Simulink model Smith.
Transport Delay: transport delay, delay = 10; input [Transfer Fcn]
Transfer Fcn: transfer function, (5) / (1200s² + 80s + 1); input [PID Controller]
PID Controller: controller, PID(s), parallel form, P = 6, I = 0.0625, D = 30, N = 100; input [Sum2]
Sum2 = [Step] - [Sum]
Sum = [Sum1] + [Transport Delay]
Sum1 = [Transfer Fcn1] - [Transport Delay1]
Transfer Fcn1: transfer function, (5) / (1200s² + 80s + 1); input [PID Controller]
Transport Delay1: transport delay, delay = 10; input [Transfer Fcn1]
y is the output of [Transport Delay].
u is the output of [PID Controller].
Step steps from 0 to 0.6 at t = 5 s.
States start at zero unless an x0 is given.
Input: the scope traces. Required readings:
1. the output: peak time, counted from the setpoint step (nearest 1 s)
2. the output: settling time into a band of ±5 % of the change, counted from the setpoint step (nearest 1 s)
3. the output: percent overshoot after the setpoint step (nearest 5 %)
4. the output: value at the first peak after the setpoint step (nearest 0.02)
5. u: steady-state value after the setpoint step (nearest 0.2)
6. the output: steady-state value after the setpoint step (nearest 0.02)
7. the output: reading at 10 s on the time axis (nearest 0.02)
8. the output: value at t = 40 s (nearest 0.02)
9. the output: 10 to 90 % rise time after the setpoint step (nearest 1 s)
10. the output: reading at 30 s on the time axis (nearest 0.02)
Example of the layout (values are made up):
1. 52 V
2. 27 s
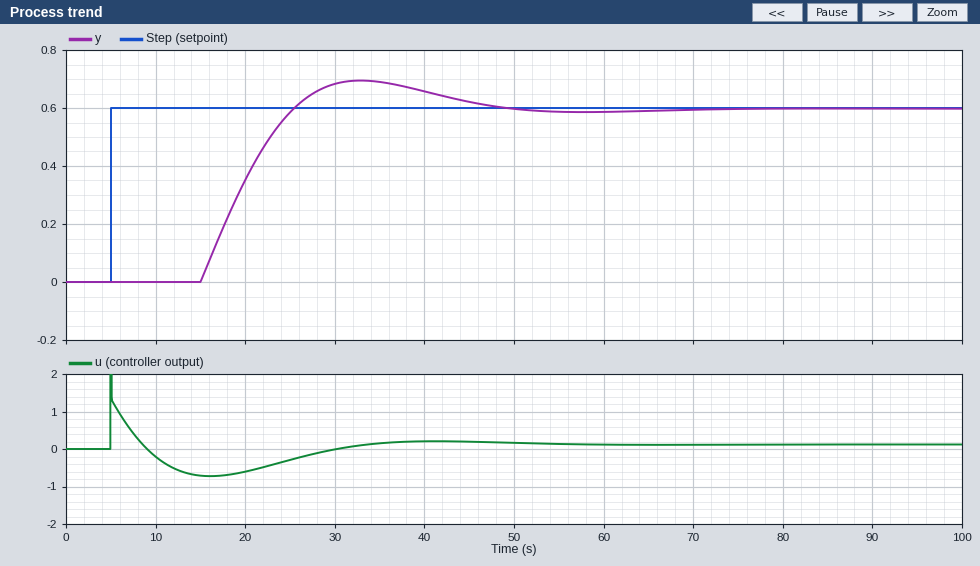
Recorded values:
1. 28 s
2. 39 s
3. 15 %
4. 0.70
5. 0.2
6. 0.60
7. 0.00
8. 0.66
9. 8 s
10. 0.68
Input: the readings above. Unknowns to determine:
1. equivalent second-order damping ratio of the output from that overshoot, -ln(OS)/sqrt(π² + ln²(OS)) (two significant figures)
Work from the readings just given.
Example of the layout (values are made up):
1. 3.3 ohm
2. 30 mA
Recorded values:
1. 0.52
